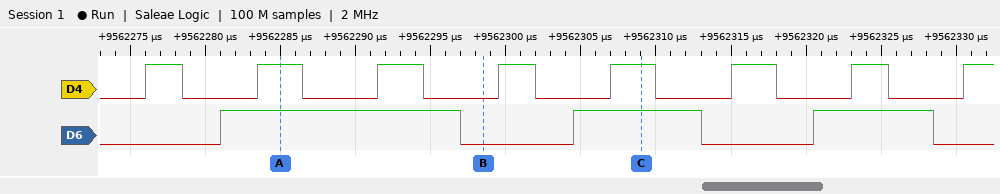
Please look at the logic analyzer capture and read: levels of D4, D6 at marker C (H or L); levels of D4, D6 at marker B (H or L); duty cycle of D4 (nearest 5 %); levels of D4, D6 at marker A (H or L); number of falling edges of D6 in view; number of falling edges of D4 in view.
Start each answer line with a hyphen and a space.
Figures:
- D4=H, D6=H
- D4=L, D6=L
- 35 %
- D4=H, D6=H
- 3
- 7
